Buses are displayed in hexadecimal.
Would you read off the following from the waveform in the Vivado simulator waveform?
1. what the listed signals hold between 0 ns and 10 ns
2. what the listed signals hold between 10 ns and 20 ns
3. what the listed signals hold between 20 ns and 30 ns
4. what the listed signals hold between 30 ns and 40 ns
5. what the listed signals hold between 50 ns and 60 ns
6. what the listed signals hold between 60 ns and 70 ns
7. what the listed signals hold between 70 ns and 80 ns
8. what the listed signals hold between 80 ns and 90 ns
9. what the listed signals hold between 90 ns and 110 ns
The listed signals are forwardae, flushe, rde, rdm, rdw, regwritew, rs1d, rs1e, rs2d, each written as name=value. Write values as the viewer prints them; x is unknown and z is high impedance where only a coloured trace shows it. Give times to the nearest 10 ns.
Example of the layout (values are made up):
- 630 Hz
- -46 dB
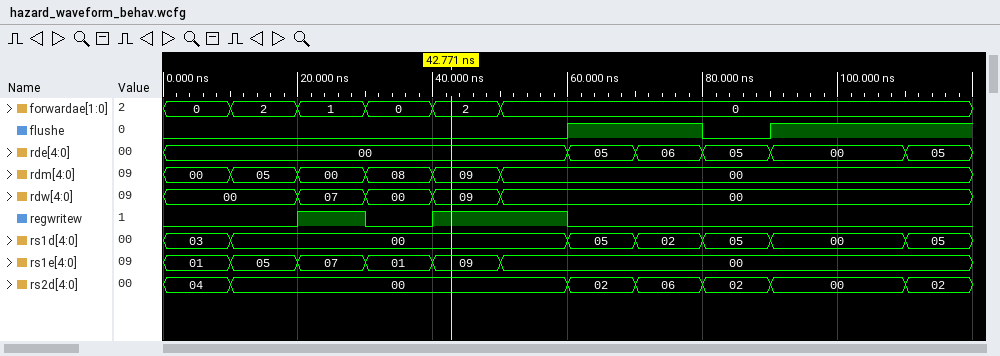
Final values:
- forwardae=0, flushe=0, rde=00, rdm=00, rdw=00, regwritew=0, rs1d=03, rs1e=01, rs2d=04
- forwardae=2, flushe=0, rde=00, rdm=05, rdw=00, regwritew=0, rs1d=00, rs1e=05, rs2d=00
- forwardae=1, flushe=0, rde=00, rdm=00, rdw=07, regwritew=1, rs1d=00, rs1e=07, rs2d=00
- forwardae=0, flushe=0, rde=00, rdm=08, rdw=00, regwritew=0, rs1d=00, rs1e=01, rs2d=00
- forwardae=0, flushe=0, rde=00, rdm=00, rdw=00, regwritew=1, rs1d=00, rs1e=00, rs2d=00
- forwardae=0, flushe=1, rde=05, rdm=00, rdw=00, regwritew=0, rs1d=05, rs1e=00, rs2d=02
- forwardae=0, flushe=1, rde=06, rdm=00, rdw=00, regwritew=0, rs1d=02, rs1e=00, rs2d=06
- forwardae=0, flushe=0, rde=05, rdm=00, rdw=00, regwritew=0, rs1d=05, rs1e=00, rs2d=02
- forwardae=0, flushe=1, rde=00, rdm=00, rdw=00, regwritew=0, rs1d=00, rs1e=00, rs2d=00
